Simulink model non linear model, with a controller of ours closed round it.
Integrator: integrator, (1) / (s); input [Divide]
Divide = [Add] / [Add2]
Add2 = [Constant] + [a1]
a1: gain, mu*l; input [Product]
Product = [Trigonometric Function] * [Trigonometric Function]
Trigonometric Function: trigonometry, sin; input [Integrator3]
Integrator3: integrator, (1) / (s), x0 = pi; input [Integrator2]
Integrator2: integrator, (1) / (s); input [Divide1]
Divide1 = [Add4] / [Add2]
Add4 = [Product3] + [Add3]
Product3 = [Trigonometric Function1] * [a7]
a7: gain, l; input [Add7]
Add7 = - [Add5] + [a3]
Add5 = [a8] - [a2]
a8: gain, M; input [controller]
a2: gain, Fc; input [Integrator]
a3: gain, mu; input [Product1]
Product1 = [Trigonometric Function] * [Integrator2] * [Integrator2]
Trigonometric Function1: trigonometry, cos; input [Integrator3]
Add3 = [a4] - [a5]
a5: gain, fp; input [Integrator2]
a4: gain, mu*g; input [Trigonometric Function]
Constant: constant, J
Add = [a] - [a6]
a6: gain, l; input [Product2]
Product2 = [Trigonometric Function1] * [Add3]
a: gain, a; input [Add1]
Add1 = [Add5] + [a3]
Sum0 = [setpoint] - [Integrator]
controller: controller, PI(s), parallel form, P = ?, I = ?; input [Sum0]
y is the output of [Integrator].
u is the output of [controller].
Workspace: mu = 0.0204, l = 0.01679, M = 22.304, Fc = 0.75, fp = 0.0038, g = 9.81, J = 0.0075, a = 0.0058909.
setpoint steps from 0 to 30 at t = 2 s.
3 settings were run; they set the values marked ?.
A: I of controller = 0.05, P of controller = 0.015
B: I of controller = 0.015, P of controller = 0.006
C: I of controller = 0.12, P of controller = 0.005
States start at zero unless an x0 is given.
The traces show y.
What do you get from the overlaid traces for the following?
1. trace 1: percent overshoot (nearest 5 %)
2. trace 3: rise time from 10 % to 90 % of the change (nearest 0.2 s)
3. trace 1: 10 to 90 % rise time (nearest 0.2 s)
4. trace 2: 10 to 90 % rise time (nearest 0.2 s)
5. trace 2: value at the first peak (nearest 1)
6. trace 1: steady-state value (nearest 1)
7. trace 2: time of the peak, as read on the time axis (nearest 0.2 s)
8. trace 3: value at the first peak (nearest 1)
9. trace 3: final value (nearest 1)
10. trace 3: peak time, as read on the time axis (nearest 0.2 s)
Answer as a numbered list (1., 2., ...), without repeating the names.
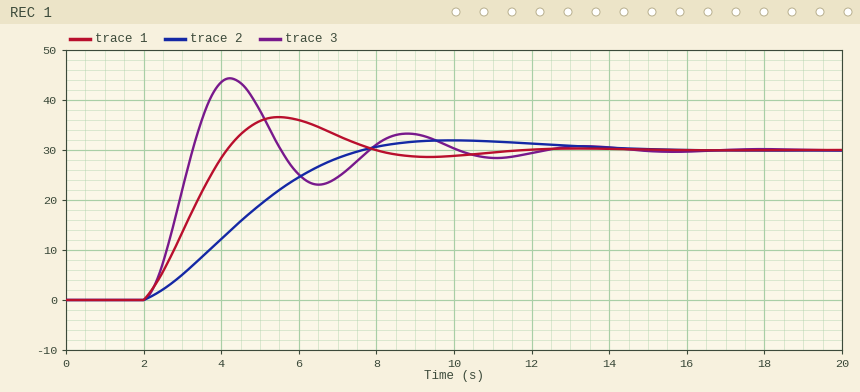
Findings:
1. 20 %
2. 0.8 s
3. 1.6 s
4. 4.0 s
5. 32
6. 30
7. 10.0 s
8. 44
9. 30
10. 4.2 s
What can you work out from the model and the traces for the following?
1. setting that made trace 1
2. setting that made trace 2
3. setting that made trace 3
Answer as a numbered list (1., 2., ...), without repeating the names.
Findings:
1. A
2. B
3. C
